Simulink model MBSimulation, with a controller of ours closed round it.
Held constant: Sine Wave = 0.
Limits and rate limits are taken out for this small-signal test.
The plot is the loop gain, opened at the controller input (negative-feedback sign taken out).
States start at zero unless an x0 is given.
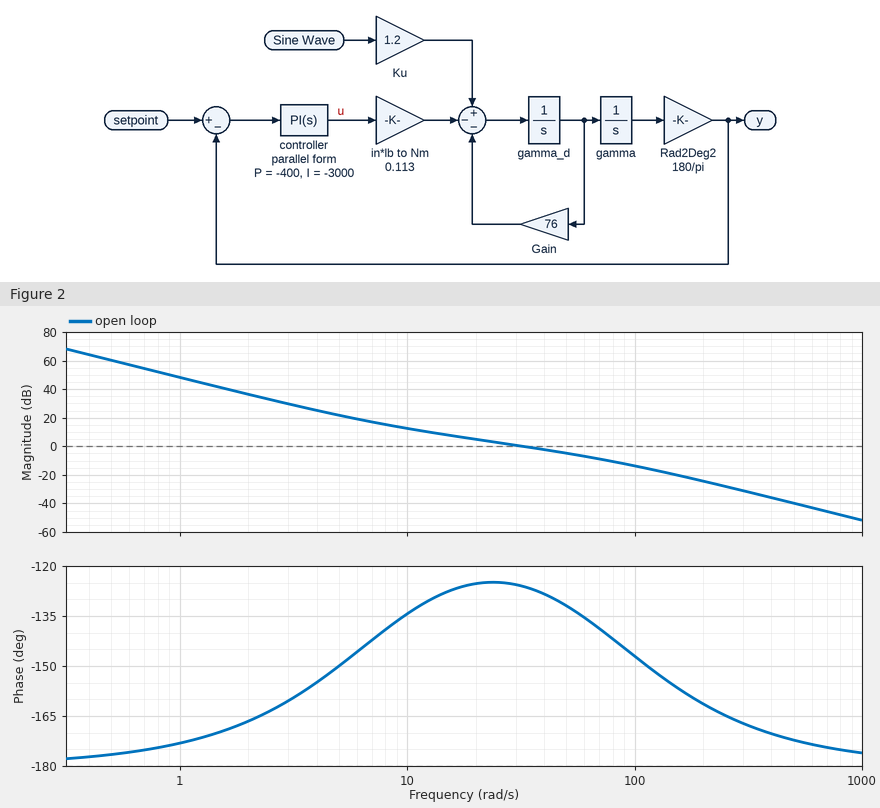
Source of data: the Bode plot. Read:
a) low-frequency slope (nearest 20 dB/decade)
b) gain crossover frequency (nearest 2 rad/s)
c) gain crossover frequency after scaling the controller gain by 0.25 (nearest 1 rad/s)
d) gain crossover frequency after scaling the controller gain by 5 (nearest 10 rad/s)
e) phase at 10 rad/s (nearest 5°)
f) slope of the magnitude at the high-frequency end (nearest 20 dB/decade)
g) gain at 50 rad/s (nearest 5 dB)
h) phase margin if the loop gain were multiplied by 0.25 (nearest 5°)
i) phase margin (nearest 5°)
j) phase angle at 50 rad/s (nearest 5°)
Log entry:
-40 dB/decade
32 rad/s
10 rad/s
100 rad/s
-135°
-40 dB/decade
-5 dB
45°
55°
-130°
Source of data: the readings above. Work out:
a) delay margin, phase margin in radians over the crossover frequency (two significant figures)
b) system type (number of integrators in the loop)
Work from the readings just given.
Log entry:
0.030 s
2
